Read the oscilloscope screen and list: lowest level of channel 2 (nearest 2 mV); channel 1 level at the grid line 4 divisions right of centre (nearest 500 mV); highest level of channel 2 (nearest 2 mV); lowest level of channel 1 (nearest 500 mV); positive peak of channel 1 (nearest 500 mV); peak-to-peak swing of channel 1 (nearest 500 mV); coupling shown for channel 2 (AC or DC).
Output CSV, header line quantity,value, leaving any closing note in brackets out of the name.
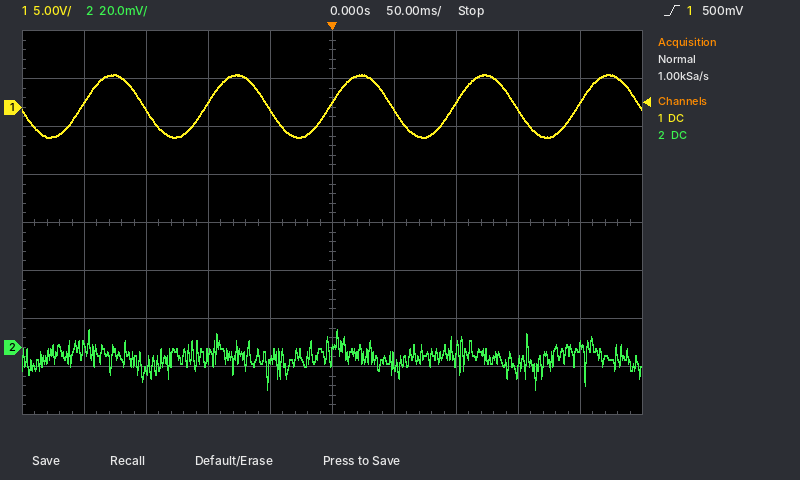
quantity,value
lowest level of channel 2,-18 mV
channel 1 level at the grid line 4 divisions right of centre,500 mV
highest level of channel 2,8 mV
lowest level of channel 1,-3.0 V
positive peak of channel 1,3.5 V
peak-to-peak swing of channel 1,6.5 V
coupling shown for channel 2,DC
